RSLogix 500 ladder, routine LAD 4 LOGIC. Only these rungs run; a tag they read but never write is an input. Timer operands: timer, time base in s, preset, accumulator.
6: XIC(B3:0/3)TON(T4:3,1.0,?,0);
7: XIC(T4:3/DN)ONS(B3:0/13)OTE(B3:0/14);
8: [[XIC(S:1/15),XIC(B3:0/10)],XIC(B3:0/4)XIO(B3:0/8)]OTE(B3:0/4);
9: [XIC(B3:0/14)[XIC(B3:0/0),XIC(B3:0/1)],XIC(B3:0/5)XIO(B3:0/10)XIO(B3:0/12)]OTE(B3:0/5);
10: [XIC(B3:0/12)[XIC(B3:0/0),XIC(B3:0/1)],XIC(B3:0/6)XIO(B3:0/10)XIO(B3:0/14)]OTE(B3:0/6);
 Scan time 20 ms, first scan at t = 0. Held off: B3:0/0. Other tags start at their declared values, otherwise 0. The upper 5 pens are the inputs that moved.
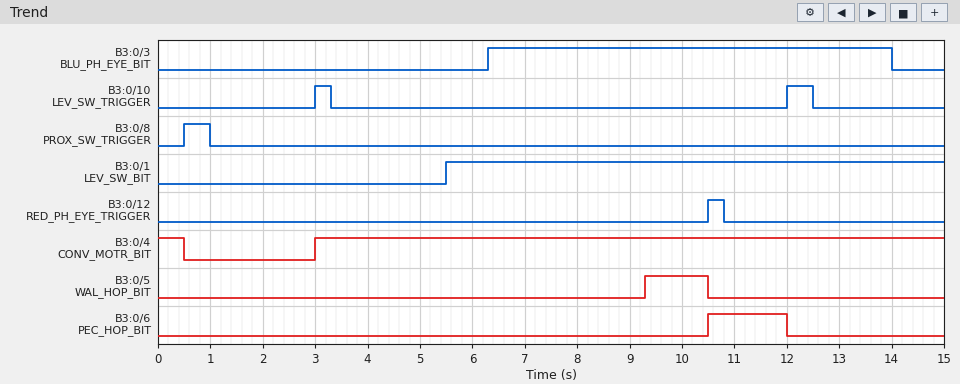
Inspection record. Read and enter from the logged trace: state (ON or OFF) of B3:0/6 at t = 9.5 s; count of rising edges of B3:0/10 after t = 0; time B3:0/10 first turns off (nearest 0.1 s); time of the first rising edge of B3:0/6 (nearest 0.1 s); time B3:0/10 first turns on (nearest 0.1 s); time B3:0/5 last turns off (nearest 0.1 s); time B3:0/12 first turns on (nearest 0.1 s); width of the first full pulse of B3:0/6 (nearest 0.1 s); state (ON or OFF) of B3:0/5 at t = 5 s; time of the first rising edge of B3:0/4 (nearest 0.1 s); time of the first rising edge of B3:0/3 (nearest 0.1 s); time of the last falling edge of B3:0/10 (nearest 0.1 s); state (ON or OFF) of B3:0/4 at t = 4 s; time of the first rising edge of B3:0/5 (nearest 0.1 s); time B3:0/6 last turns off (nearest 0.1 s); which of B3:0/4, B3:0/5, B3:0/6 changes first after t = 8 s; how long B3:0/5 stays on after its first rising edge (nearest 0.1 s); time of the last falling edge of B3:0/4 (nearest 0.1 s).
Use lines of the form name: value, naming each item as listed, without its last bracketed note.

state (ON or OFF) of B3:0/6 at t = 9.5 s: OFF
count of rising edges of B3:0/10 after t = 0: 2
time B3:0/10 first turns off: 3.3 s
time of the first rising edge of B3:0/6: 10.5 s
time B3:0/10 first turns on: 3.0 s
time B3:0/5 last turns off: 10.5 s
time B3:0/12 first turns on: 10.5 s
width of the first full pulse of B3:0/6: 1.5 s
state (ON or OFF) of B3:0/5 at t = 5 s: OFF
time of the first rising edge of B3:0/4: 3.0 s
time of the first rising edge of B3:0/3: 6.3 s
time of the last falling edge of B3:0/10: 12.5 s
state (ON or OFF) of B3:0/4 at t = 4 s: ON
time of the first rising edge of B3:0/5: 9.3 s
time B3:0/6 last turns off: 12.0 s
which of B3:0/4, B3:0/5, B3:0/6 changes first after t = 8 s: B3:0/5
how long B3:0/5 stays on after its first rising edge: 1.2 s
time of the last falling edge of B3:0/4: 0.5 s
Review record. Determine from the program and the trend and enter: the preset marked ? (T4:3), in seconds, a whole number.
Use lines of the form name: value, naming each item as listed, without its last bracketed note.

the preset marked ? (T4:3), in seconds, a whole number: 3 s
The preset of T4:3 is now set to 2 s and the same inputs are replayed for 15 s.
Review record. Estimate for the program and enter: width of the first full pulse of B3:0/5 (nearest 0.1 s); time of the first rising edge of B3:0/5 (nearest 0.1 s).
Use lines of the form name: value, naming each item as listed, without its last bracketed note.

width of the first full pulse of B3:0/5: 2.2 s
time of the first rising edge of B3:0/5: 8.3 s
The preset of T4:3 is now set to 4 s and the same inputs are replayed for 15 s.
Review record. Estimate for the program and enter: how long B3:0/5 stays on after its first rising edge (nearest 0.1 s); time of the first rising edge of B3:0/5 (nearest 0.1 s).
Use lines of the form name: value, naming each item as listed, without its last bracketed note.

how long B3:0/5 stays on after its first rising edge: 0.2 s
time of the first rising edge of B3:0/5: 10.3 s
